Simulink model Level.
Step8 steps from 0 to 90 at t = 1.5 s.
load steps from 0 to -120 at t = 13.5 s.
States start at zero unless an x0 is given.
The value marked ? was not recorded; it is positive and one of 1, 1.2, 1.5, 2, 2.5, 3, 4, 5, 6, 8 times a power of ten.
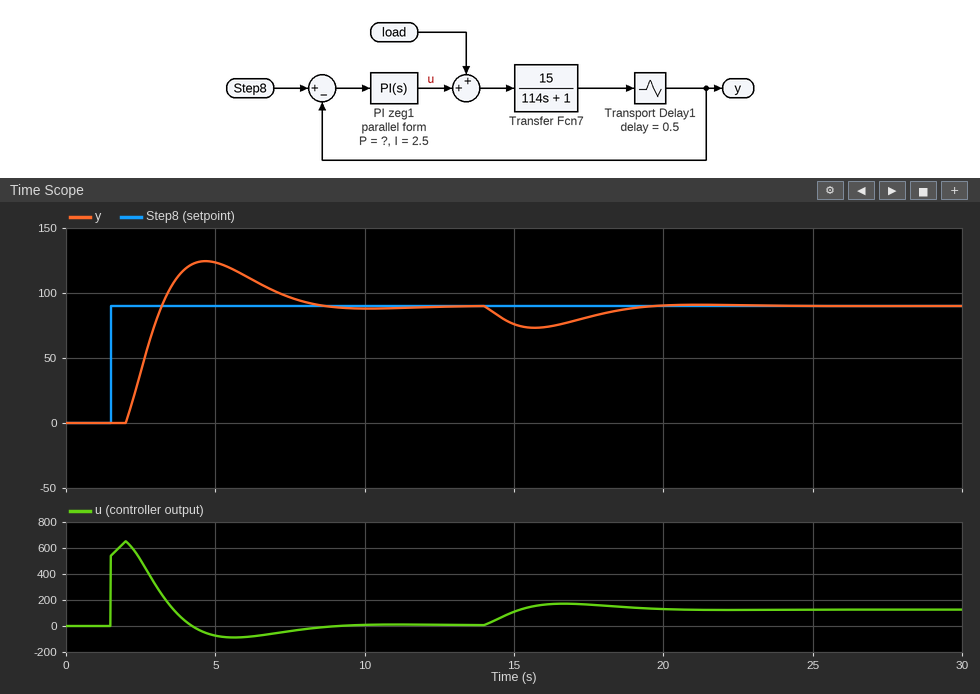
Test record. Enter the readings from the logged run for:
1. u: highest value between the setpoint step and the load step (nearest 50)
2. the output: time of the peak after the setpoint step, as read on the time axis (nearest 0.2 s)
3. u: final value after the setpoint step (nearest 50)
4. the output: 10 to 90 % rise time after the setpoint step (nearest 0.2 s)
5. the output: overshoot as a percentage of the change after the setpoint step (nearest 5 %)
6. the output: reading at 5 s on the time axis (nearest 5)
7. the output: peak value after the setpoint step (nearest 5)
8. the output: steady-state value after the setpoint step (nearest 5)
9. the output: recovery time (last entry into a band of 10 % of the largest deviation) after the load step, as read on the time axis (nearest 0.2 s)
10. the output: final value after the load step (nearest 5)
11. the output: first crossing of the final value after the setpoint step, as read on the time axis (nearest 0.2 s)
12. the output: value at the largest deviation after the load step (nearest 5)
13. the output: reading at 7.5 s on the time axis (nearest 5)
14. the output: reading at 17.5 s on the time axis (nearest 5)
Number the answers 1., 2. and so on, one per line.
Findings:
1. 650
2. 4.6 s
3. 0
4. 1.0 s
5. 40 %
6. 125
7. 125
8. 90
9. 19.0 s
10. 90
11. 3.2 s
12. 75
13. 95
14. 80
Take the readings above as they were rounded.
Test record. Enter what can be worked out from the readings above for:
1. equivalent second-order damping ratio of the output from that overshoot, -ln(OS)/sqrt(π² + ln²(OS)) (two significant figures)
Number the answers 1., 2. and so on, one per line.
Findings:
1. 0.28
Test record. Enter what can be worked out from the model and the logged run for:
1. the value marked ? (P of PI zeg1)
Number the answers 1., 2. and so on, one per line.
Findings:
1. 6
